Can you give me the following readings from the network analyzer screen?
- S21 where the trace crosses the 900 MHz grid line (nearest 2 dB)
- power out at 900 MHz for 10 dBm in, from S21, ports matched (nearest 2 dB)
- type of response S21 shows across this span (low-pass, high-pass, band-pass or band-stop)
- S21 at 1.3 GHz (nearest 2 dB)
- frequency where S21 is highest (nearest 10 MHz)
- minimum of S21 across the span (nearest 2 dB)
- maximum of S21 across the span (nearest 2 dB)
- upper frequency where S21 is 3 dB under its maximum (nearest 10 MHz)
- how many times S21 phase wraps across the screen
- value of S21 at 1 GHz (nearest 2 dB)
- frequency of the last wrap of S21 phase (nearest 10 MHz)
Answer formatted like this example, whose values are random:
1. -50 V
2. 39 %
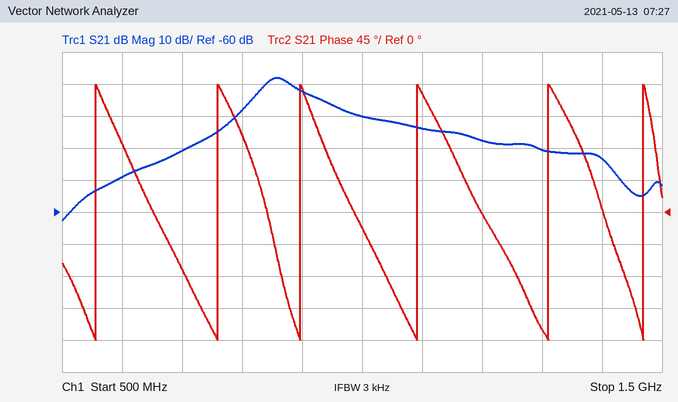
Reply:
1. -22 dB
2. -12 dBm
3. band-pass
4. -40 dB
5. 860 MHz
6. -62 dB
7. -18 dB
8. 890 MHz
9. 6
10. -30 dB
11. 1.47 GHz
